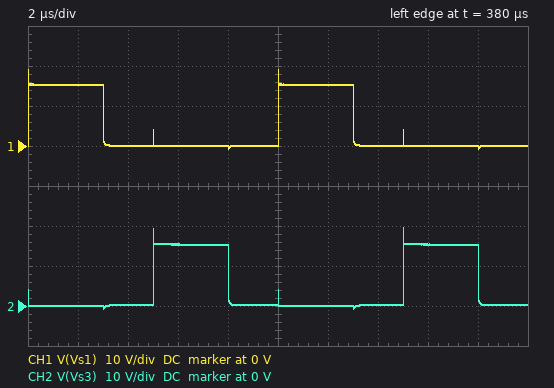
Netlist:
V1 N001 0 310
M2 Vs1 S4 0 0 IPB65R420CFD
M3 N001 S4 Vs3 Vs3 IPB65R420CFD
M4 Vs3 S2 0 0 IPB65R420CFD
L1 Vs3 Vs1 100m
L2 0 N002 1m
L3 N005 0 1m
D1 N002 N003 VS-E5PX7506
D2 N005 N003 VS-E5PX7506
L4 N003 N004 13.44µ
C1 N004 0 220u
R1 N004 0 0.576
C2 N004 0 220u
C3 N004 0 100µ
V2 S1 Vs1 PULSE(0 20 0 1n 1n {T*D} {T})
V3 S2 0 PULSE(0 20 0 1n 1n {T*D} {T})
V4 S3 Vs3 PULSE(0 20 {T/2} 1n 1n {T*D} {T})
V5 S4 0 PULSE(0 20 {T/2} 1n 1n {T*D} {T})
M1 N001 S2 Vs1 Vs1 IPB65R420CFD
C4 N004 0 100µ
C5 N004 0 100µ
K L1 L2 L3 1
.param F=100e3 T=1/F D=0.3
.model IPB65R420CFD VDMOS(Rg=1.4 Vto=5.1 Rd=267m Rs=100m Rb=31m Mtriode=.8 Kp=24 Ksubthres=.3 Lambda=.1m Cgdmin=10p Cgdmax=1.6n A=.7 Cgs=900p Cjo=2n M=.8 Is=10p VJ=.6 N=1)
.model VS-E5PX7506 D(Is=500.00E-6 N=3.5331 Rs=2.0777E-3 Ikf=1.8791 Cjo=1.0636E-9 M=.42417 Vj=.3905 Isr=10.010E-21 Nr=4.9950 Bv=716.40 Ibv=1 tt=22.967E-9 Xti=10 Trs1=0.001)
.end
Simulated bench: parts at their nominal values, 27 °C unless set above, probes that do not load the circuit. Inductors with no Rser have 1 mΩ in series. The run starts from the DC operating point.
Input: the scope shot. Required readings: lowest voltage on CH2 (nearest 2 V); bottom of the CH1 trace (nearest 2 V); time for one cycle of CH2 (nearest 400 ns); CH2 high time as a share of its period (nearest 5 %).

0 V
0 V
10.0 µs
30 %
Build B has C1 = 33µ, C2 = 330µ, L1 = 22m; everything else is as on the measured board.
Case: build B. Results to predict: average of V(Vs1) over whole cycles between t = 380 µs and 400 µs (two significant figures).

4.5 V
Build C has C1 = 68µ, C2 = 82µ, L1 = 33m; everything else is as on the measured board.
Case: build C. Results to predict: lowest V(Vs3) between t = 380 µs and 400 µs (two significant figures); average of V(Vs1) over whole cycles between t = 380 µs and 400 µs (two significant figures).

-700 mV
4.5 V
